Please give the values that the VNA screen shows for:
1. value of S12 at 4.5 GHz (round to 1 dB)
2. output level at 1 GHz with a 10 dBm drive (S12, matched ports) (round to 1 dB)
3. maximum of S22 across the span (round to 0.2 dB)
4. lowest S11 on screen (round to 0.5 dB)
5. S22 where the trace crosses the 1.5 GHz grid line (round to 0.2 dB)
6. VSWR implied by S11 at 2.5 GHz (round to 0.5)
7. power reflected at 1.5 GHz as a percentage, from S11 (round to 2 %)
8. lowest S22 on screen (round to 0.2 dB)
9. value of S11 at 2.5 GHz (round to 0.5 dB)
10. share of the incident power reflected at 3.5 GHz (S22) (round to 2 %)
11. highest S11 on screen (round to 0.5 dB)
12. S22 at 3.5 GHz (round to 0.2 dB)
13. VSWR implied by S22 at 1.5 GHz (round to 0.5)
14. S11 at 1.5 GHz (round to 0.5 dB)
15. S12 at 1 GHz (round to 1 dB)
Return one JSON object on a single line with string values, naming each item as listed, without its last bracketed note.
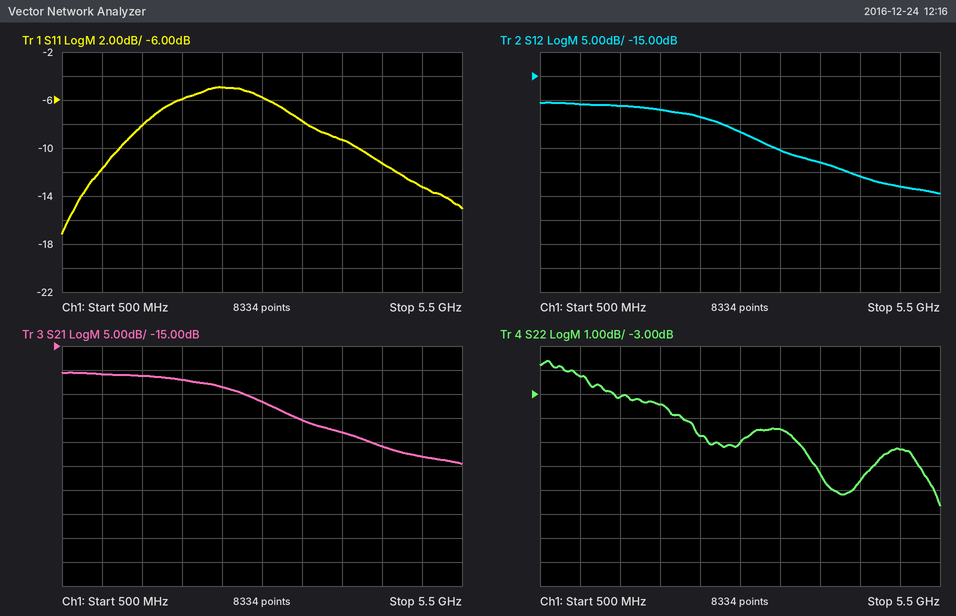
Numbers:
{"value of S12 at 4.5 GHz": "-36 dB", "output level at 1 GHz with a 10 dBm drive (S12, matched ports)": "-11 dBm", "maximum of S22 across the span": "-1.6 dB", "lowest S11 on screen": "-17.0 dB", "S22 where the trace crosses the 1.5 GHz grid line": "-3.2 dB", "VSWR implied by S11 at 2.5 GHz": "3.5", "power reflected at 1.5 GHz as a percentage, from S11": "16 %", "lowest S22 on screen": "-7.6 dB", "value of S11 at 2.5 GHz": "-5.0 dB", "share of the incident power reflected at 3.5 GHz (S22)": "36 %", "highest S11 on screen": "-5.0 dB", "S22 at 3.5 GHz": "-4.4 dB", "VSWR implied by S22 at 1.5 GHz": "5.5", "S11 at 1.5 GHz": "-8.0 dB", "S12 at 1 GHz": "-21 dB"}
